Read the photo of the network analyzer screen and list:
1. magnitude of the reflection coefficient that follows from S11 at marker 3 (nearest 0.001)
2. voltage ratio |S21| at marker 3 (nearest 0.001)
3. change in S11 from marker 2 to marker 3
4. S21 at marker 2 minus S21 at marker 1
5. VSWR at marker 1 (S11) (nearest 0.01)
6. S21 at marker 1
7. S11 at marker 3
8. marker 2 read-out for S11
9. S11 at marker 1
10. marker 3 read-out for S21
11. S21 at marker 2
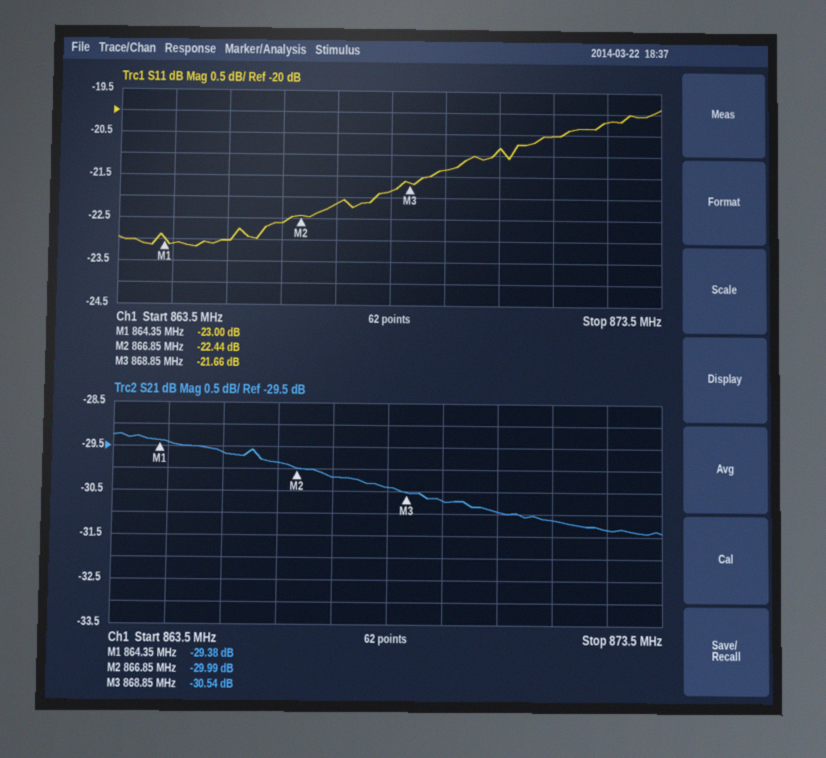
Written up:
0.083
0.030
0.78 dB
-0.61 dB
1.15
-29.38 dB
-21.66 dB
-22.44 dB
-23.00 dB
-30.54 dB
-29.99 dB
